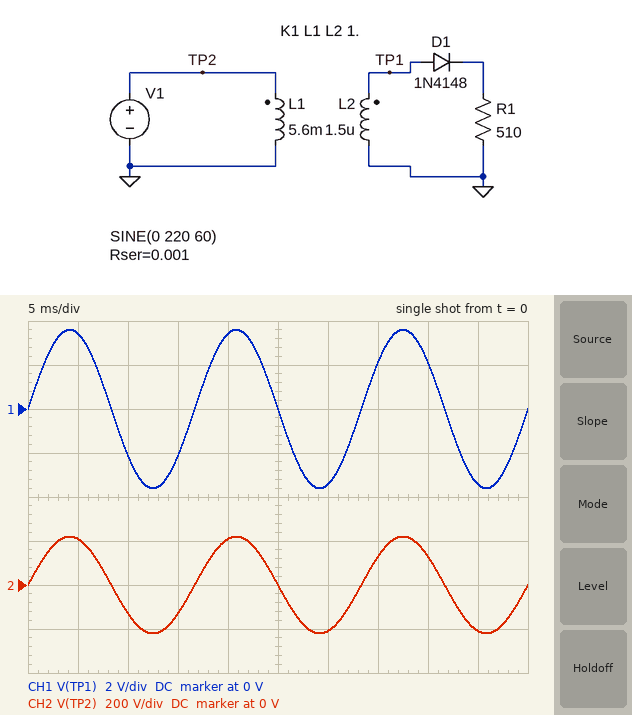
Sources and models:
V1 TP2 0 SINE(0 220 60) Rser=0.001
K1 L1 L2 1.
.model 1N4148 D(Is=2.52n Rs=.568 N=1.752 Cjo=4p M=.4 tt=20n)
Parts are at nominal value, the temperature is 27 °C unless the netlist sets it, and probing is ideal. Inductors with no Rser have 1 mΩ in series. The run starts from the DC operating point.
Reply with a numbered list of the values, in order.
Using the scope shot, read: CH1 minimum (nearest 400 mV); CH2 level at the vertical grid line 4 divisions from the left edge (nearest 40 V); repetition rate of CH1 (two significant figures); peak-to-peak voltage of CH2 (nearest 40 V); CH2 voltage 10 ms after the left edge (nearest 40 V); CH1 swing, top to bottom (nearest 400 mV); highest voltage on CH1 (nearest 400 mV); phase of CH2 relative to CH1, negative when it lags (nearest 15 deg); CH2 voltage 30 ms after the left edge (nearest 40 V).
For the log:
1. -3.6 V
2. 200 V
3. 60 Hz
4. 440 V
5. -120 V
6. 7.2 V
7. 3.6 V
8. 0 deg
9. -200 V
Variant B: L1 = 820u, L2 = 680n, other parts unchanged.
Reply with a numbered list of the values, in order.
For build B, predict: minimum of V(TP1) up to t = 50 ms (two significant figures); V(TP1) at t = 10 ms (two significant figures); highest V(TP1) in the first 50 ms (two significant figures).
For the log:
1. -6.4 V
2. -3.8 V
3. 6.3 V
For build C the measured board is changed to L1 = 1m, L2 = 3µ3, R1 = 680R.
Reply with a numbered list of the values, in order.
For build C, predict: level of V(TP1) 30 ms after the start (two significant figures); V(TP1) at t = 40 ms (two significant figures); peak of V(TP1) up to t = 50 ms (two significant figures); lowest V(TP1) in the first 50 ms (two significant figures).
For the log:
1. -12 V
2. 7.3 V
3. 13 V
4. -13 V
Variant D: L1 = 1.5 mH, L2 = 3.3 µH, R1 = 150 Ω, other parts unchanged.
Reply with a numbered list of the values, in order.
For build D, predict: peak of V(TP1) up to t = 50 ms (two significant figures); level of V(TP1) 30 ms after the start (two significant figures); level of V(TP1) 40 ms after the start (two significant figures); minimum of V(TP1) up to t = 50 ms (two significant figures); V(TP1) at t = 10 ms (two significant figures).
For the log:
1. 10 V
2. -9.8 V
3. 6.0 V
4. -10 V
5. -6.1 V
